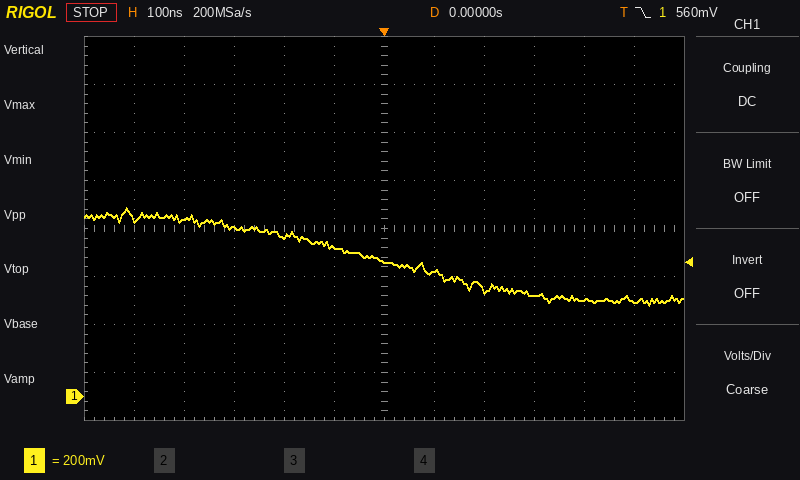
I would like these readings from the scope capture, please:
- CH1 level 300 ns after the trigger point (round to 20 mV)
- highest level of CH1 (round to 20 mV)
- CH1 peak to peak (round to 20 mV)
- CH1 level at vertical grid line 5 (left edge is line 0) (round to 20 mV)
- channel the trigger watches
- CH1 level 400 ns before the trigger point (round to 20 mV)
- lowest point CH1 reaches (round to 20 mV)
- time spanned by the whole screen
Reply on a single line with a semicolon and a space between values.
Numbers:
420 mV; 780 mV; 400 mV; 620 mV; CH1; 740 mV; 380 mV; 1.2 µs
